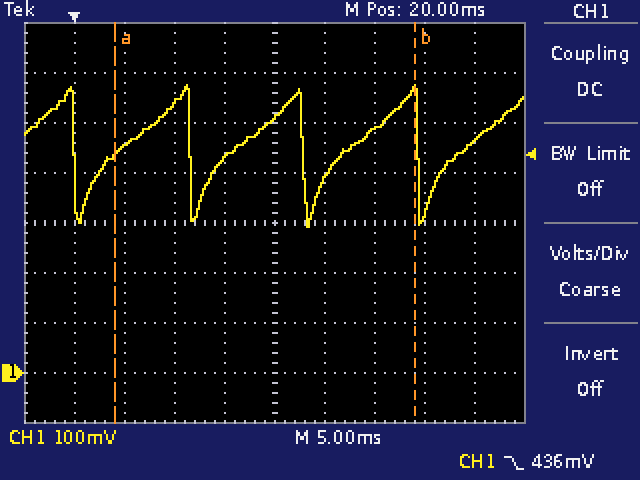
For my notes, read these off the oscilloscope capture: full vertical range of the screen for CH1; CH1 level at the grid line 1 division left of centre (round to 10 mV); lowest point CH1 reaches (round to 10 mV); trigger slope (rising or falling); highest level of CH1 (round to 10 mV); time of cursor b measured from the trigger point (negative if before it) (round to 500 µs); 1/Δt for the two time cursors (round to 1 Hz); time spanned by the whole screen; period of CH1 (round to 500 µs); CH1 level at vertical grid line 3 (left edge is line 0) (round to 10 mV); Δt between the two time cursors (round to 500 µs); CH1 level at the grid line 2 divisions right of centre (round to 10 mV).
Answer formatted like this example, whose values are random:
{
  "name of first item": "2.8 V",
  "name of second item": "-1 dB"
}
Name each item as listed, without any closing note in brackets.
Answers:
{
  "full vertical range of the screen for CH1": "800 mV",
  "CH1 level at the grid line 1 division left of centre": "430 mV",
  "lowest point CH1 reaches": "290 mV",
  "trigger slope": "falling",
  "highest level of CH1": "580 mV",
  "time of cursor b measured from the trigger point (negative if before it)": "+34.0 ms",
  "1/Δt for the two time cursors": "33 Hz",
  "time spanned by the whole screen": "50 ms",
  "period of CH1": "11.5 ms",
  "CH1 level at vertical grid line 3 (left edge is line 0)": "540 mV",
  "Δt between the two time cursors": "30.0 ms",
  "CH1 level at the grid line 2 divisions right of centre": "490 mV"
}
